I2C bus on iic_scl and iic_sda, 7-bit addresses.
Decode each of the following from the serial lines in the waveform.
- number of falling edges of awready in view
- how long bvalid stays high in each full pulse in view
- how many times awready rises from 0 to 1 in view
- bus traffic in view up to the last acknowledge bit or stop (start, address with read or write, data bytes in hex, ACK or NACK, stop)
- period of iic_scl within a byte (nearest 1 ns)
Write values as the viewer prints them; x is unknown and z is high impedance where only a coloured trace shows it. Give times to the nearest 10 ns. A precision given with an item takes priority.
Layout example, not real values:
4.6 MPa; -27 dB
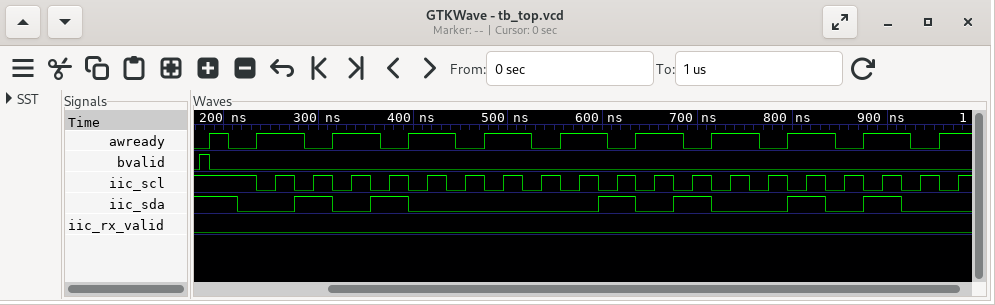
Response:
10; 10 ns; 11; start, address 28 write ACK, A5 ACK; 40 ns
